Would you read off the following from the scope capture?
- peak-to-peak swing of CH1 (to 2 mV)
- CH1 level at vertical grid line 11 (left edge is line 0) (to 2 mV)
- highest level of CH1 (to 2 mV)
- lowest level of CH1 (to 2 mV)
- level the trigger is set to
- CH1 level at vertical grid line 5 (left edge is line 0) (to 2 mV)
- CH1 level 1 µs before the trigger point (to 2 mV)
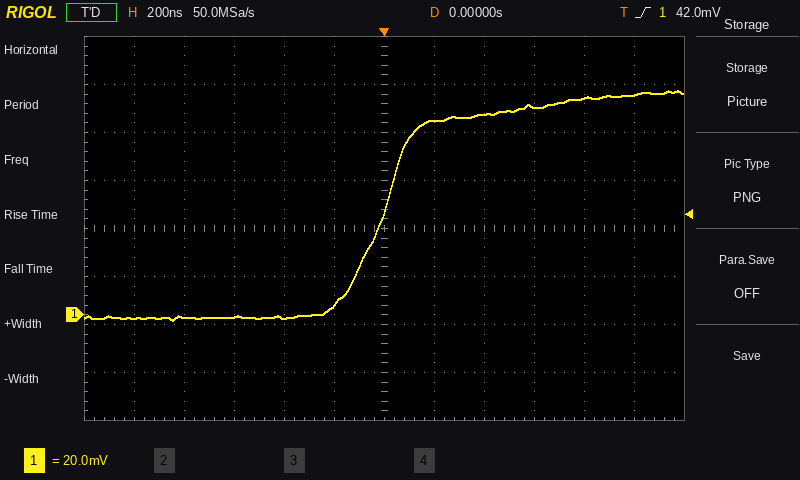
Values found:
96 mV
92 mV
94 mV
-2 mV
42.0 mV
4 mV
-2 mV
